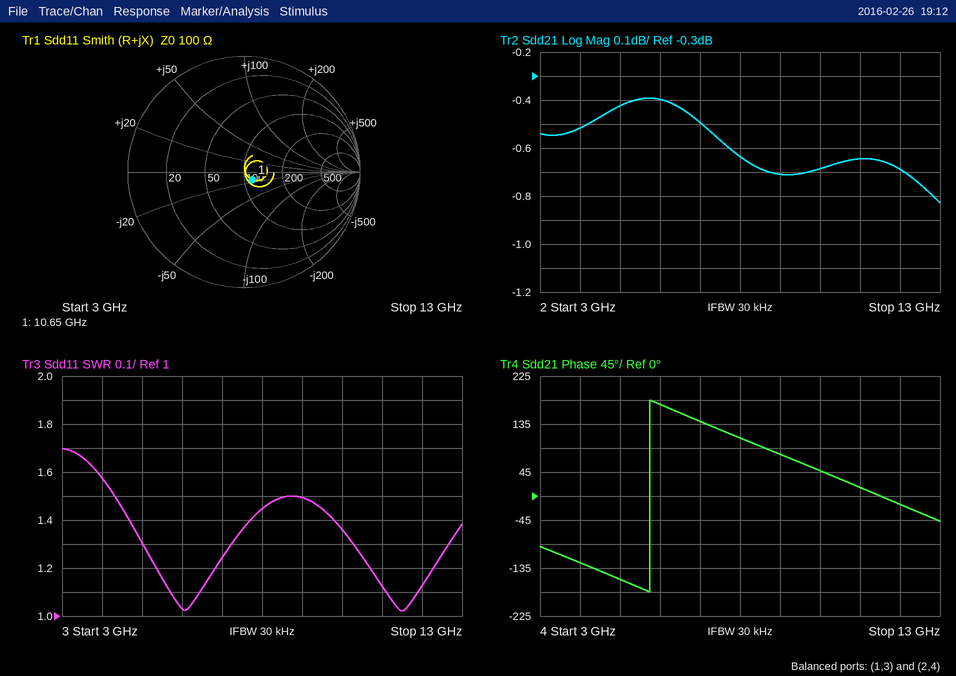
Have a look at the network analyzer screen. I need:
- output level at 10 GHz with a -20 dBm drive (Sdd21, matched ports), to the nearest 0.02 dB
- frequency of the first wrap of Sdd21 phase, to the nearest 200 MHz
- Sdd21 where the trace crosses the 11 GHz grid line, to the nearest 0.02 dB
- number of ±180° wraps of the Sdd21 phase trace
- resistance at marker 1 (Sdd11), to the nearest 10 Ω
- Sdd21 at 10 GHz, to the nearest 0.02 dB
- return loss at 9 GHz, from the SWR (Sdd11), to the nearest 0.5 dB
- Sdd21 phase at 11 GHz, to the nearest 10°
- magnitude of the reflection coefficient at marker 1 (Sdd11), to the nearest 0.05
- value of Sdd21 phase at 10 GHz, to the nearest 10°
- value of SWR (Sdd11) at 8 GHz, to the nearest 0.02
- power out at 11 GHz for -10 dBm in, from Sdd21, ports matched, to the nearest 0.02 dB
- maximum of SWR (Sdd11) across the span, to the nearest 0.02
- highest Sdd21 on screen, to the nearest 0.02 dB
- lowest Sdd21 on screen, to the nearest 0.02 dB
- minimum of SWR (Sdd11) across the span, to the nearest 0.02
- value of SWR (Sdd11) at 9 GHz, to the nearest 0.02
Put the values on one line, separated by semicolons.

-20.68 dBm; 5.8 GHz; -0.64 dB; 1; 110 Ω; -0.68 dB; 14.0 dB; 20°; 0.10; 50°; 1.44; -10.64 dBm; 1.70; -0.40 dB; -0.82 dB; 1.02; 1.50
